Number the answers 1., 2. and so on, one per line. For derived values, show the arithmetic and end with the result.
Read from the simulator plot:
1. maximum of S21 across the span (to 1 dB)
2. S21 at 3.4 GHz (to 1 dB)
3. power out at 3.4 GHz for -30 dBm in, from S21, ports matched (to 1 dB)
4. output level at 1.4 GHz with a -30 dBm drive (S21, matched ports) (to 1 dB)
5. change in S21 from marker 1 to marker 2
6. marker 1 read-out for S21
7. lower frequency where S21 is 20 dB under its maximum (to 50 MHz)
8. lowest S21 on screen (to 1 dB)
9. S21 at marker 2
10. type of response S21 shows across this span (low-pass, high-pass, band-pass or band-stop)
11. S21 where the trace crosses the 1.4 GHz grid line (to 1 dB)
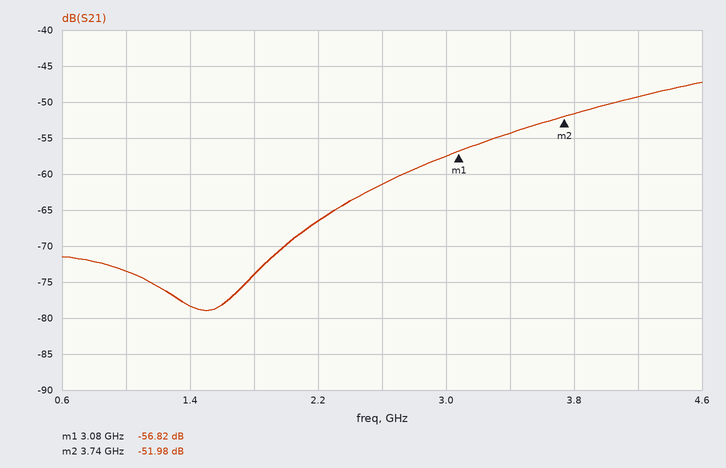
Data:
1. -47 dB
2. -54 dB
3. -30 dBm + (-54 dB) = -84 dBm
4. -30 dBm + (-78 dB) = -108 dBm
5. -51.98 − (-56.82) = 4.84 dB
6. -56.82 dB
7. 2.15 GHz
8. -79 dB
9. -51.98 dB
10. high-pass
11. -78 dB
